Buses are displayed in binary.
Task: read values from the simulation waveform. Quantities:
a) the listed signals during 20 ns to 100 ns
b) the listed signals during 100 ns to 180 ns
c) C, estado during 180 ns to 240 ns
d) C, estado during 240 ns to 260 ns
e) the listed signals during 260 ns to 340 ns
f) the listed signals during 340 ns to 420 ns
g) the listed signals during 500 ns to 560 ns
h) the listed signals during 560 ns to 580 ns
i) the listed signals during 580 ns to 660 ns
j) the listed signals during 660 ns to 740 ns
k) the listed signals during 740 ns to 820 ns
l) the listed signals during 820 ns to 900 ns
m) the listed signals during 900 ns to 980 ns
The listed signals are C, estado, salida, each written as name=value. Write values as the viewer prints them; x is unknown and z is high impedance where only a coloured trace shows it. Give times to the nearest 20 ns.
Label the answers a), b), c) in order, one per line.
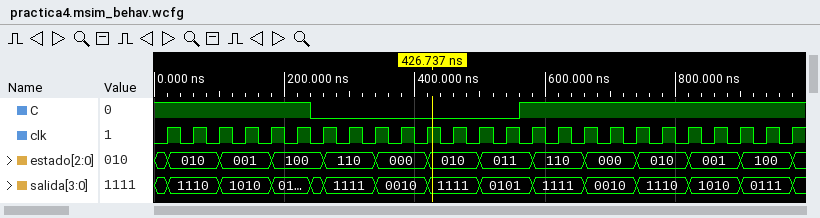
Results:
a) C=1, estado=010, salida=1110
b) C=1, estado=001, salida=1010
c) C=1, estado=100
d) C=0, estado=100
e) C=0, estado=110, salida=1111
f) C=0, estado=000, salida=0010
g) C=0, estado=011, salida=0101
h) C=1, estado=011, salida=0101
i) C=1, estado=110, salida=1111
j) C=1, estado=000, salida=0010
k) C=1, estado=010, salida=1110
l) C=1, estado=001, salida=1010
m) C=1, estado=100, salida=0111
